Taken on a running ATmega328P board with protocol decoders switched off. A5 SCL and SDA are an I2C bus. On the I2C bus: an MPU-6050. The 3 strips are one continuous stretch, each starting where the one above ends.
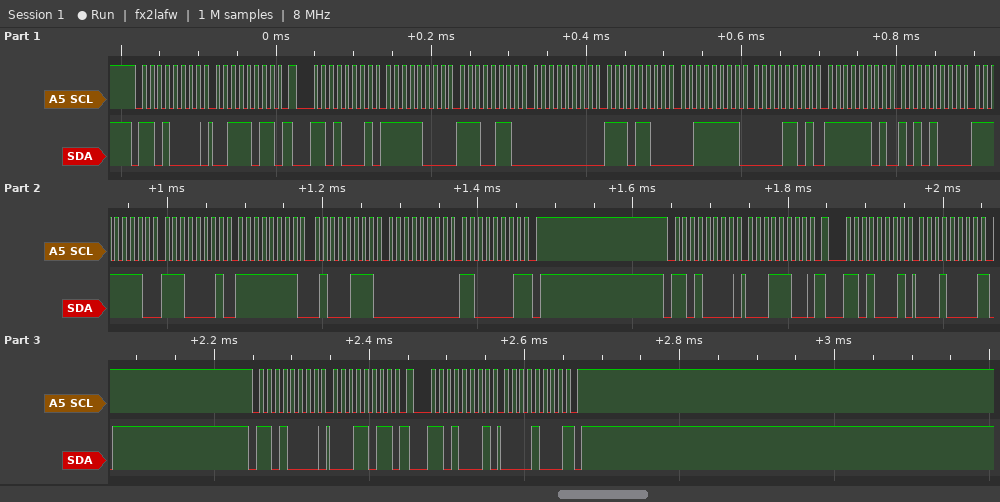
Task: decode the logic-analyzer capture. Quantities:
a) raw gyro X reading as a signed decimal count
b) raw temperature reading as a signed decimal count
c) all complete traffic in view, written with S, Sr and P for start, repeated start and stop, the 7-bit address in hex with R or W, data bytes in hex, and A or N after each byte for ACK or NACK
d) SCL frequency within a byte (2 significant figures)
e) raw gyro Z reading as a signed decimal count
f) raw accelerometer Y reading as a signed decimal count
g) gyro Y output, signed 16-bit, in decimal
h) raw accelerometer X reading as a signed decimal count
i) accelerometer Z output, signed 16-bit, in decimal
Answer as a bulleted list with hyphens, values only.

- -287
- -600
- S 68W A 3B A Sr 68R A F8 A E6 A 00 A EC A 3F A 0D A FD A A8 A FE A E1 A FF A 47 A 00 A C1 N P S 68W A 1C A Sr 68R A 10 N P S 68W A 1B A Sr 68R A 08 N P
- 100 kHz
- 193
- 236
- -185
- -1818
- 16141
